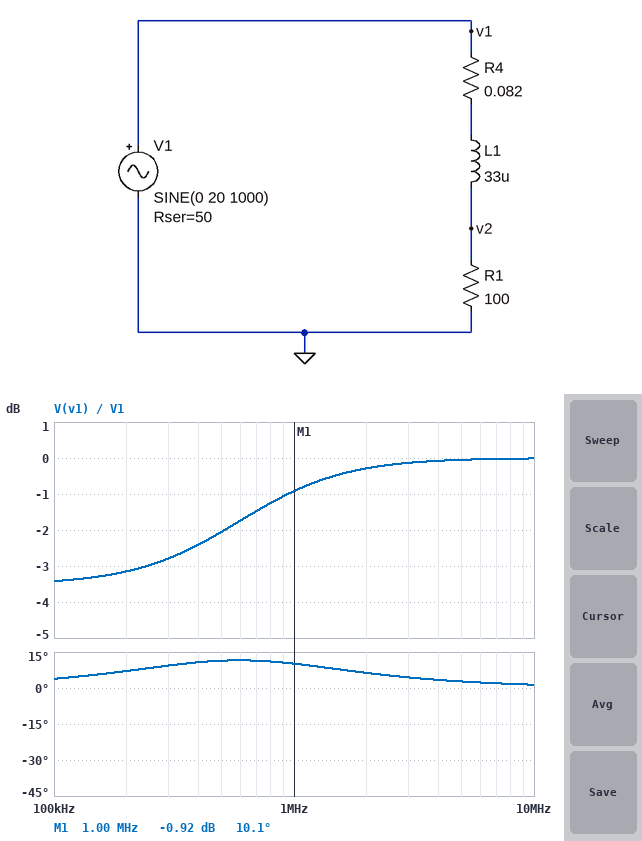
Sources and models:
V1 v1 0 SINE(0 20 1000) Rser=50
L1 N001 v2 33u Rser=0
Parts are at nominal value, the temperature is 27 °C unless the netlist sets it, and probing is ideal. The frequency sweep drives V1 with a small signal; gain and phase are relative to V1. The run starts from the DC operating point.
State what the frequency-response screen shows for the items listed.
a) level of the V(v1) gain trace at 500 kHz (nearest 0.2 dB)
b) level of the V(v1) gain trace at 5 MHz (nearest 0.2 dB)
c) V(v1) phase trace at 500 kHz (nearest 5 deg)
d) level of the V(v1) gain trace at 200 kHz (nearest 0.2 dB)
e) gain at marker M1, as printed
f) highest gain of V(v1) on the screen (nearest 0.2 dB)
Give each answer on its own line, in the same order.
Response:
-2.0 dB
0 dB
10 deg
-3.2 dB
-0.92 dB
0 dB
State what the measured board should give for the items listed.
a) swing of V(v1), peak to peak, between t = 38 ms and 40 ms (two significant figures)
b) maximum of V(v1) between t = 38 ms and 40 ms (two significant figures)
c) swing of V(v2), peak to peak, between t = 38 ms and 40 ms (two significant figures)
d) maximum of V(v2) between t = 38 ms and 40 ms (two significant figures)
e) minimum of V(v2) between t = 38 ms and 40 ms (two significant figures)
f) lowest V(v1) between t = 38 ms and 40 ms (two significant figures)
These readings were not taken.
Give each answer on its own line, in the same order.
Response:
27 V
13 V
27 V
13 V
-13 V
-13 V
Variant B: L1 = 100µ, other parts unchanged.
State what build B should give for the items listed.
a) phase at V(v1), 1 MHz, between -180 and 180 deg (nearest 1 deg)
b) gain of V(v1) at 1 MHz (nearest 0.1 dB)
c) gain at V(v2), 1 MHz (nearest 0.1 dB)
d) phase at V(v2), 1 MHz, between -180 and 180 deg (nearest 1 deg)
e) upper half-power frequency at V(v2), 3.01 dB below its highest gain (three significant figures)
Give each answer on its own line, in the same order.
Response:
4 deg
-0.1 dB
-16.2 dB
-77 deg
239 kHz
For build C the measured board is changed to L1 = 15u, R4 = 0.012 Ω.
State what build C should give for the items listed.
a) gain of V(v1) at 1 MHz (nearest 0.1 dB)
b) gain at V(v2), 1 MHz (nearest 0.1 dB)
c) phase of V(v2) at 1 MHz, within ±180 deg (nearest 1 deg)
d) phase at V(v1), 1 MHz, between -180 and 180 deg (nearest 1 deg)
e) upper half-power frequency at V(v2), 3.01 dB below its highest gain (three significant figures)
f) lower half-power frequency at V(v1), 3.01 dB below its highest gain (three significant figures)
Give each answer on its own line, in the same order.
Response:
-2.2 dB
-5.0 dB
-32 deg
11 deg
1.59 MHz
530 kHz
